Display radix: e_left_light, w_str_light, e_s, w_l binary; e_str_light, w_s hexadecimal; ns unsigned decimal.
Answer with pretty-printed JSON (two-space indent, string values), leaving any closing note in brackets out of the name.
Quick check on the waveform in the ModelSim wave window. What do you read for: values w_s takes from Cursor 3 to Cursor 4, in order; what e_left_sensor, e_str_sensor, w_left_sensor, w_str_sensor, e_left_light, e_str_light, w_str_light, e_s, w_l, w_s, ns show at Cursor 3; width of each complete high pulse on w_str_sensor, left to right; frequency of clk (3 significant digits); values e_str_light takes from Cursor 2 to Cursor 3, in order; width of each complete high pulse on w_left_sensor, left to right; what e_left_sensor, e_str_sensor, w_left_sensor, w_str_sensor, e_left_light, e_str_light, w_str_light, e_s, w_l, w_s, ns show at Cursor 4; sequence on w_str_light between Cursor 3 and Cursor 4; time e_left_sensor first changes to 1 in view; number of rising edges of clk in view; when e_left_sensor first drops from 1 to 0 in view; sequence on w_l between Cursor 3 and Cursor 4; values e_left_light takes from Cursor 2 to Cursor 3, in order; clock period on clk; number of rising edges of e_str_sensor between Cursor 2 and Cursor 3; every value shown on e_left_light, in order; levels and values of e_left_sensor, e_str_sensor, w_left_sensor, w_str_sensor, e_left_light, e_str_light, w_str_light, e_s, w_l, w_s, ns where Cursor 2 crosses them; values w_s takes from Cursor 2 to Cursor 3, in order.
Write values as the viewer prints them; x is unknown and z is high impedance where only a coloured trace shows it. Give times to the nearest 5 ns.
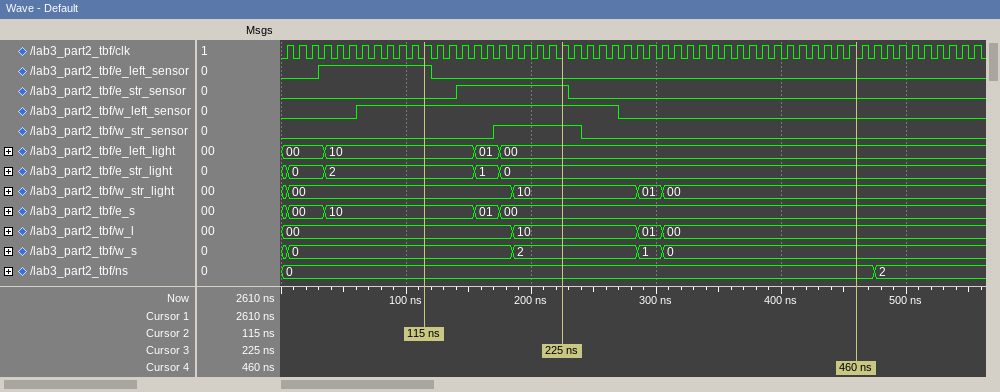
{
  "values w_s takes from Cursor 3 to Cursor 4, in order": "2, 1, 0",
  "what e_left_sensor, e_str_sensor, w_left_sensor, w_str_sensor, e_left_light, e_str_light, w_str_light, e_s, w_l, w_s, ns show at Cursor 3": "e_left_sensor=0, e_str_sensor=1, w_left_sensor=1, w_str_sensor=1, e_left_light=00, e_str_light=0, w_str_light=10, e_s=00, w_l=10, w_s=2, ns=0",
  "width of each complete high pulse on w_str_sensor, left to right": "70 ns",
  "frequency of clk": "100 MHz",
  "values e_str_light takes from Cursor 2 to Cursor 3, in order": "2, 1, 0",
  "width of each complete high pulse on w_left_sensor, left to right": "210 ns",
  "what e_left_sensor, e_str_sensor, w_left_sensor, w_str_sensor, e_left_light, e_str_light, w_str_light, e_s, w_l, w_s, ns show at Cursor 4": "e_left_sensor=0, e_str_sensor=0, w_left_sensor=0, w_str_sensor=0, e_left_light=00, e_str_light=0, w_str_light=00, e_s=00, w_l=00, w_s=0, ns=0",
  "sequence on w_str_light between Cursor 3 and Cursor 4": "10, 01, 00",
  "time e_left_sensor first changes to 1 in view": "30 ns",
  "number of rising edges of clk in view": "56",
  "when e_left_sensor first drops from 1 to 0 in view": "120 ns",
  "sequence on w_l between Cursor 3 and Cursor 4": "10, 01, 00",
  "values e_left_light takes from Cursor 2 to Cursor 3, in order": "10, 01, 00",
  "clock period on clk": "10 ns",
  "number of rising edges of e_str_sensor between Cursor 2 and Cursor 3": "1",
  "every value shown on e_left_light, in order": "00, 10, 01, 00",
  "levels and values of e_left_sensor, e_str_sensor, w_left_sensor, w_str_sensor, e_left_light, e_str_light, w_str_light, e_s, w_l, w_s, ns where Cursor 2 crosses them": "e_left_sensor=1, e_str_sensor=0, w_left_sensor=1, w_str_sensor=0, e_left_light=10, e_str_light=2, w_str_light=00, e_s=10, w_l=00, w_s=0, ns=0",
  "values w_s takes from Cursor 2 to Cursor 3, in order": "0, 2"
}
